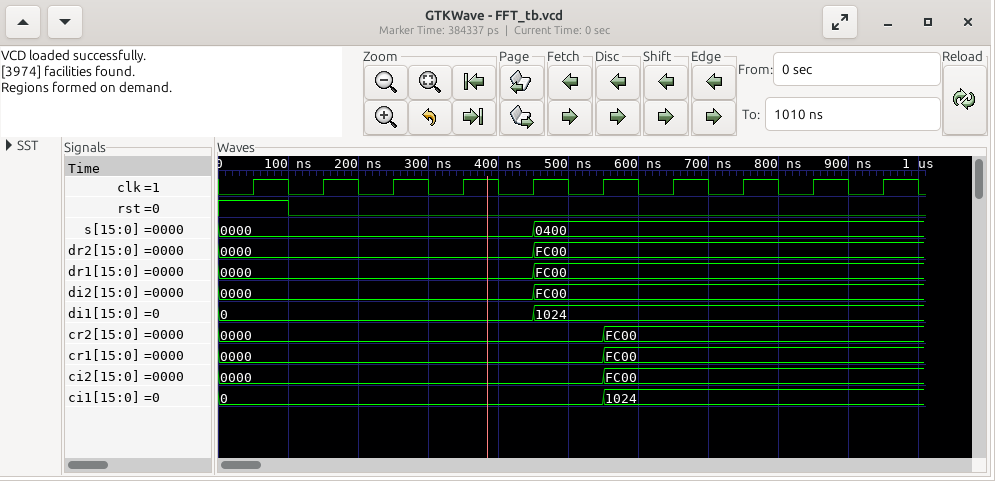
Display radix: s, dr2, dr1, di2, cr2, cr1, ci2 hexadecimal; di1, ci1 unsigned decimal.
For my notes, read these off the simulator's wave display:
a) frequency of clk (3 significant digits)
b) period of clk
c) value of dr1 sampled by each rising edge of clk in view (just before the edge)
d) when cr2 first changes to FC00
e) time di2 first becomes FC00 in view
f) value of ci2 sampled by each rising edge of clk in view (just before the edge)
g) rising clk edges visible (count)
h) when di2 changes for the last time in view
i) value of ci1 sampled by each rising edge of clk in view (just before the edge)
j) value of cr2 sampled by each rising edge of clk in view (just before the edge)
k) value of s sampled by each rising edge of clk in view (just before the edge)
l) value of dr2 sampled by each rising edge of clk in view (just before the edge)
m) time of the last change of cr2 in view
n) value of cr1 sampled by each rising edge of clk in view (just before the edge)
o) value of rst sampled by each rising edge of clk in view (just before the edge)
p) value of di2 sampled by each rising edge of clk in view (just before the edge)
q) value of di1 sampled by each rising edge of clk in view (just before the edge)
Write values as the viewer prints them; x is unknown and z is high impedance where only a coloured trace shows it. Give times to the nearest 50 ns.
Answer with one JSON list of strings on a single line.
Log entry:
["10.0 MHz", "100 ns", "0000, 0000, 0000, 0000, 0000, FC00, FC00, FC00, FC00, FC00", "550 ns", "450 ns", "0000, 0000, 0000, 0000, 0000, 0000, FC00, FC00, FC00, FC00", "10", "450 ns", "0, 0, 0, 0, 0, 0, 1024, 1024, 1024, 1024", "0000, 0000, 0000, 0000, 0000, 0000, FC00, FC00, FC00, FC00", "0000, 0000, 0000, 0000, 0000, 0400, 0400, 0400, 0400, 0400", "0000, 0000, 0000, 0000, 0000, FC00, FC00, FC00, FC00, FC00", "550 ns", "0000, 0000, 0000, 0000, 0000, 0000, FC00, FC00, FC00, FC00", "1 0 0 0 0 0 0 0 0 0", "0000, 0000, 0000, 0000, 0000, FC00, FC00, FC00, FC00, FC00", "0, 0, 0, 0, 0, 1024, 1024, 1024, 1024, 1024"]
